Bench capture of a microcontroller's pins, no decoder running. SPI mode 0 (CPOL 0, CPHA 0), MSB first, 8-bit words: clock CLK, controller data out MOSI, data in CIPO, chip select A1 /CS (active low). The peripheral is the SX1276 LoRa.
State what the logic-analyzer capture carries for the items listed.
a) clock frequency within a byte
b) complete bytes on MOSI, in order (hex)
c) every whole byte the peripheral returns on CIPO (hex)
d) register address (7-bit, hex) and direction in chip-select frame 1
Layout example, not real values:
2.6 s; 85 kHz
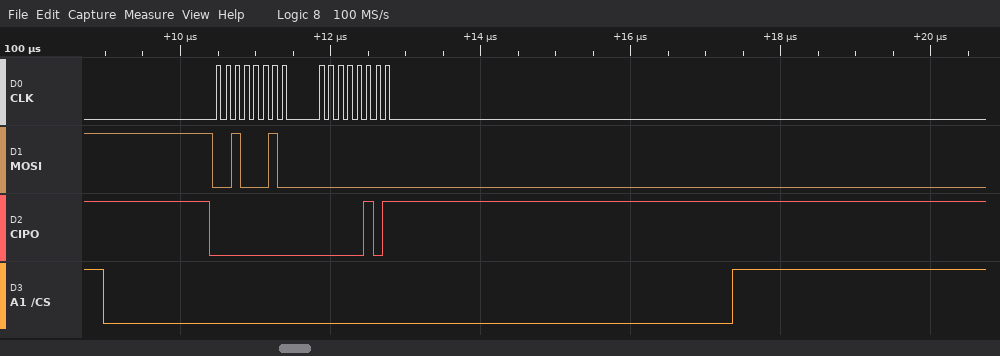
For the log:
8 MHz; 0x22 0x00; 0x00 0x05; 0x22 read
